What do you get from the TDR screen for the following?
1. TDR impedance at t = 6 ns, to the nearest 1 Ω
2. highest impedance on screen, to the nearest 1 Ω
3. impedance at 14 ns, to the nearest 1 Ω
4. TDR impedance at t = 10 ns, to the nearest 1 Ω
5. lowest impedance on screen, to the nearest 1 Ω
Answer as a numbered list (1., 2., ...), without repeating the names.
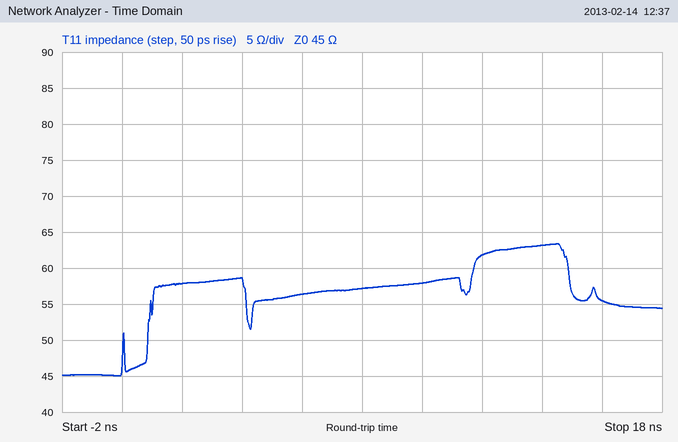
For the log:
1. 56 Ω
2. 63 Ω
3. 63 Ω
4. 58 Ω
5. 45 Ω
